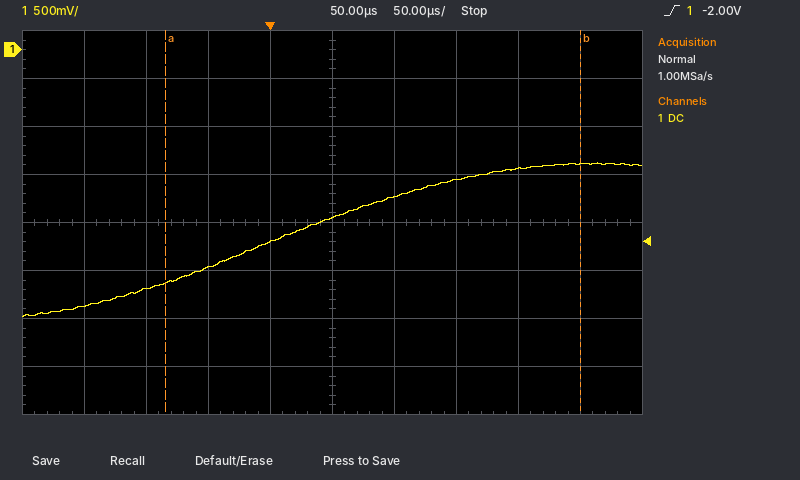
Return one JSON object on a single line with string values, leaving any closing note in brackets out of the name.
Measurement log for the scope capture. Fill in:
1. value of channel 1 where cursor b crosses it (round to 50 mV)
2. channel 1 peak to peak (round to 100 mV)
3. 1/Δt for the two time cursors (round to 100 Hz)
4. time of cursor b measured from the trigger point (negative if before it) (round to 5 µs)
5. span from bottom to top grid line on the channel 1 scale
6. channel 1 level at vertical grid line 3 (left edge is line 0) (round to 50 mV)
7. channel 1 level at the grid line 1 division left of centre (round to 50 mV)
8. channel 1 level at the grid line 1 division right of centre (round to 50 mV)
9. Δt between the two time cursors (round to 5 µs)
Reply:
{"value of channel 1 where cursor b crosses it": "-1.20 V", "channel 1 peak to peak": "1.60 V", "1/Δt for the two time cursors": "3.0 kHz", "time of cursor b measured from the trigger point (negative if before it)": "+250 µs", "span from bottom to top grid line on the channel 1 scale": "4 V", "channel 1 level at vertical grid line 3 (left edge is line 0)": "-2.25 V", "channel 1 level at the grid line 1 division left of centre": "-2.00 V", "channel 1 level at the grid line 1 division right of centre": "-1.55 V", "Δt between the two time cursors": "335 µs"}
